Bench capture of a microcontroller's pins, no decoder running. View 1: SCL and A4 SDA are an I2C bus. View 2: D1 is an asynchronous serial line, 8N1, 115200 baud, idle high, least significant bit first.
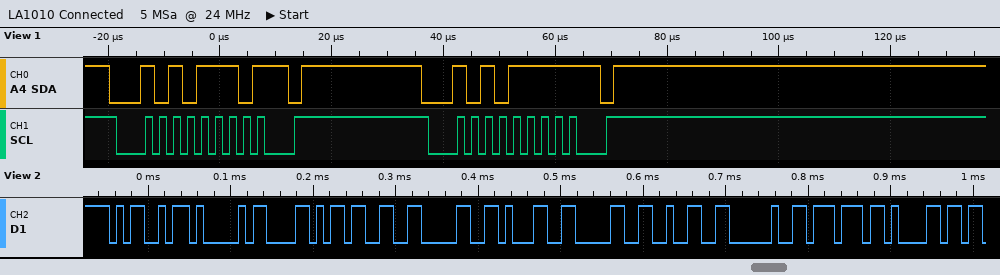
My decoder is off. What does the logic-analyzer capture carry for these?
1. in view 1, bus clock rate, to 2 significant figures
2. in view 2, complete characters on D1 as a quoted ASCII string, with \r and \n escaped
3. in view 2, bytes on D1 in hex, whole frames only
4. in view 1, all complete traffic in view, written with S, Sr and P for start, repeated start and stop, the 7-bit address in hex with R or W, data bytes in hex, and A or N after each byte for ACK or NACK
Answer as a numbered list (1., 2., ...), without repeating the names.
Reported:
1. 400 kHz
2. "MAX30102 wa"
3. 4D 41 58 33 30 31 30 32 20 77 61
4. S 57W N P S 57R N P
